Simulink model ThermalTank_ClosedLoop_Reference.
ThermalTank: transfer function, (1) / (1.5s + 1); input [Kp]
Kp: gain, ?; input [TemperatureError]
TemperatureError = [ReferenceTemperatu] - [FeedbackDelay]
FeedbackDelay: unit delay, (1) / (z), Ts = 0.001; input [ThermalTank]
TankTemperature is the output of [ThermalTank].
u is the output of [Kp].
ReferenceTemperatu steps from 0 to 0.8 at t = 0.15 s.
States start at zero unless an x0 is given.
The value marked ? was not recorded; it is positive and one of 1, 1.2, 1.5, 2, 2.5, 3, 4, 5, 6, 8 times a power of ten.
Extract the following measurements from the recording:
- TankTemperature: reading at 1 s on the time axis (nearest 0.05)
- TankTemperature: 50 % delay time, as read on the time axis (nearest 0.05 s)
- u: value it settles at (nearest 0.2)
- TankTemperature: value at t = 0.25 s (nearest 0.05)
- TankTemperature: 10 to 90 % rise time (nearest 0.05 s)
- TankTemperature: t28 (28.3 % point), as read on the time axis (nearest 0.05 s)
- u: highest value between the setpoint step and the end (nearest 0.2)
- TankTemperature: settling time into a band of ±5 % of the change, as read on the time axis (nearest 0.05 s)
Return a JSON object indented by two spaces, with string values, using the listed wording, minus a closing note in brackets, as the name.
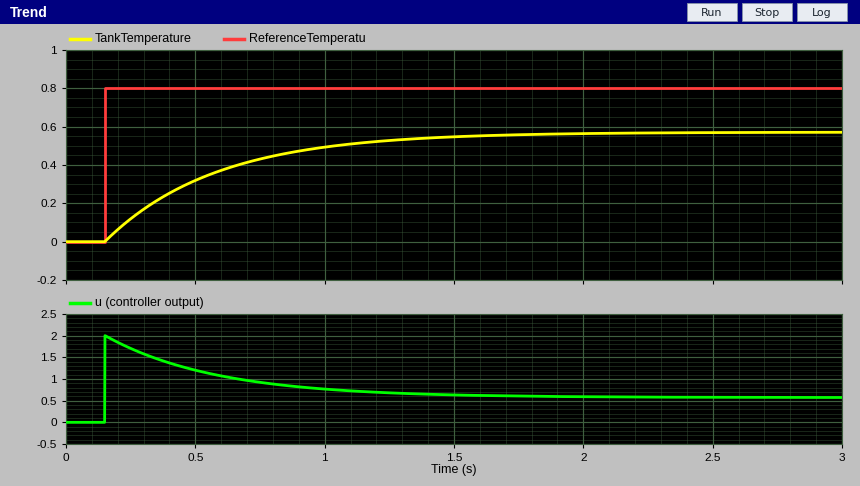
{
  "TankTemperature: reading at 1 s on the time axis": "0.50",
  "TankTemperature: 50 % delay time, as read on the time axis": "0.45 s",
  "u: value it settles at": "0.6",
  "TankTemperature: value at t = 0.25 s": "0.10",
  "TankTemperature: 10 to 90 % rise time": "0.95 s",
  "TankTemperature: t28 (28.3 % point), as read on the time axis": "0.30 s",
  "u: highest value between the setpoint step and the end": "2.0",
  "TankTemperature: settling time into a band of ±5 % of the change, as read on the time axis": "1.45 s"
}
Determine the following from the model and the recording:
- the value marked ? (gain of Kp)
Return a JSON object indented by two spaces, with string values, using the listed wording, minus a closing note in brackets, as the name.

{
  "the value marked ?": "2.5"
}
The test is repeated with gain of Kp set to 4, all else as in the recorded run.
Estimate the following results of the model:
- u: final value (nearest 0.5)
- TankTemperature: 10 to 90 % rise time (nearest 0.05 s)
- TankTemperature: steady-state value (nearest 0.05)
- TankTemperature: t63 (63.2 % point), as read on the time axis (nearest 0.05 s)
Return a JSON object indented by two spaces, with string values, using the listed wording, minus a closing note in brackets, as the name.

{
  "u: final value": "0.5",
  "TankTemperature: 10 to 90 % rise time": "0.65 s",
  "TankTemperature: steady-state value": "0.65",
  "TankTemperature: t63 (63.2 % point), as read on the time axis": "0.45 s"
}
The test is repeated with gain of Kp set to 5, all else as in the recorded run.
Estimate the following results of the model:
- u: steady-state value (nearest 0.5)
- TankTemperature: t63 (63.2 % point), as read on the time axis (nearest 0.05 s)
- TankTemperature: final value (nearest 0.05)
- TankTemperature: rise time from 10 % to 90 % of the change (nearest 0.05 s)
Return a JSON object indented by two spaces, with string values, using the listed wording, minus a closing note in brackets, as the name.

{
  "u: steady-state value": "0.5",
  "TankTemperature: t63 (63.2 % point), as read on the time axis": "0.40 s",
  "TankTemperature: final value": "0.65",
  "TankTemperature: rise time from 10 % to 90 % of the change": "0.55 s"
}
